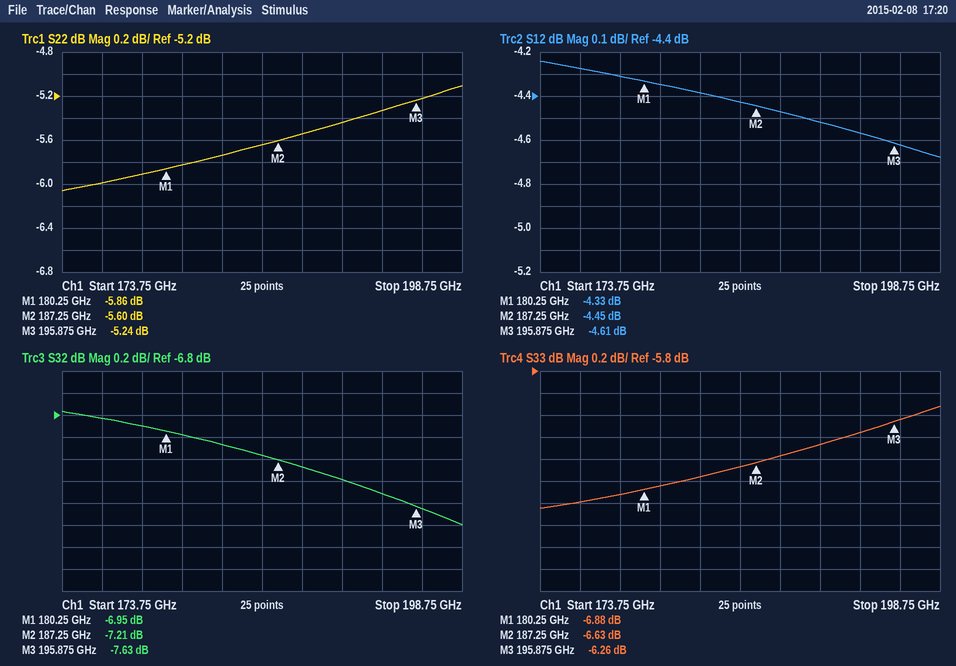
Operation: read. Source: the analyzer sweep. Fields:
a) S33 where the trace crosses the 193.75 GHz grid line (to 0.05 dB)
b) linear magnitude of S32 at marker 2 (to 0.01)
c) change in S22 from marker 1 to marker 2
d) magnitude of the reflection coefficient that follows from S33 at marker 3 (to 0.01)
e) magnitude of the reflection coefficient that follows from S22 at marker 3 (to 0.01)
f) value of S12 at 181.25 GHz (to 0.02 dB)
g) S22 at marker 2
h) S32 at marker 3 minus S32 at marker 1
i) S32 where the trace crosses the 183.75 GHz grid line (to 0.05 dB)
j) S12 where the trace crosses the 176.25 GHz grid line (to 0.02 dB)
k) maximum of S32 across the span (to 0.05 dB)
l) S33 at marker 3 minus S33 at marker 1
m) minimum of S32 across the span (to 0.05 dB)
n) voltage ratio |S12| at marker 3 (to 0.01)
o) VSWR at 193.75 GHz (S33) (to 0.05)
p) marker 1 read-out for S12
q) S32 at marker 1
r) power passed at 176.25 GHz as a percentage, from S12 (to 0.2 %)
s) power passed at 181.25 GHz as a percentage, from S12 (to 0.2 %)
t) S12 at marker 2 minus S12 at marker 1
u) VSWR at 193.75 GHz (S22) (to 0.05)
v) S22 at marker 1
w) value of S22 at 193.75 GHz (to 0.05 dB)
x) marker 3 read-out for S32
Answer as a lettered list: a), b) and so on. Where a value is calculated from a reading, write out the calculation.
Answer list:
a) -6.35 dB
b) 10^(-7.21/20) ≈ 0.44
c) -5.6 − (-5.86) = 0.26 dB
d) 10^(-6.26/20) ≈ 0.49
e) 10^(-5.24/20) ≈ 0.55
f) -4.34 dB
g) -5.60 dB
h) -7.63 − (-6.95) = -0.68 dB
i) -7.05 dB
j) -4.28 dB
k) -6.75 dB
l) -6.26 − (-6.88) = 0.62 dB
m) -7.80 dB
n) 10^(-4.61/20) ≈ 0.59
o) |Γ| = 10^(-6.35/20) = 0.4814; VSWR = (1 + 0.4814)/(1 − 0.4814) ≈ 2.86, so 2.85 to the nearest 0.05
p) -4.33 dB
q) -6.95 dB
r) 10^(-4.28/10) ≈ 37.3 %, so 37.4 % to the nearest 0.2 %
s) 10^(-4.34/10) ≈ 36.8 %
t) -4.45 − (-4.33) = -0.12 dB
u) |Γ| = 10^(-5.35/20) = 0.5401; VSWR = (1 + 0.5401)/(1 − 0.5401) ≈ 3.35
v) -5.86 dB
w) -5.35 dB
x) -7.63 dB
